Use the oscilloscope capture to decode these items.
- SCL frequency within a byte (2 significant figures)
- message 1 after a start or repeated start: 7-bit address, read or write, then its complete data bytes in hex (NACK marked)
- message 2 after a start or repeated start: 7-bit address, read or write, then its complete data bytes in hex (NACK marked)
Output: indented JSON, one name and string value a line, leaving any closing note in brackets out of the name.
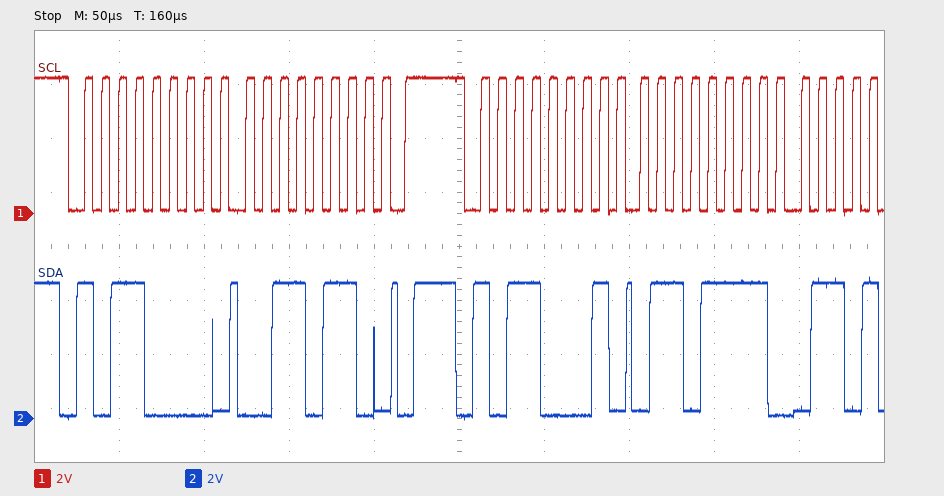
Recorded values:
{
  "SCL frequency within a byte": "100 kHz",
  "message 1 after a start or repeated start: 7-bit address, read or write, then its complete data bytes in hex": "0x58 write: 36",
  "message 2 after a start or repeated start: 7-bit address, read or write, then its complete data bytes in hex": "0x58 read: 6F"
}
